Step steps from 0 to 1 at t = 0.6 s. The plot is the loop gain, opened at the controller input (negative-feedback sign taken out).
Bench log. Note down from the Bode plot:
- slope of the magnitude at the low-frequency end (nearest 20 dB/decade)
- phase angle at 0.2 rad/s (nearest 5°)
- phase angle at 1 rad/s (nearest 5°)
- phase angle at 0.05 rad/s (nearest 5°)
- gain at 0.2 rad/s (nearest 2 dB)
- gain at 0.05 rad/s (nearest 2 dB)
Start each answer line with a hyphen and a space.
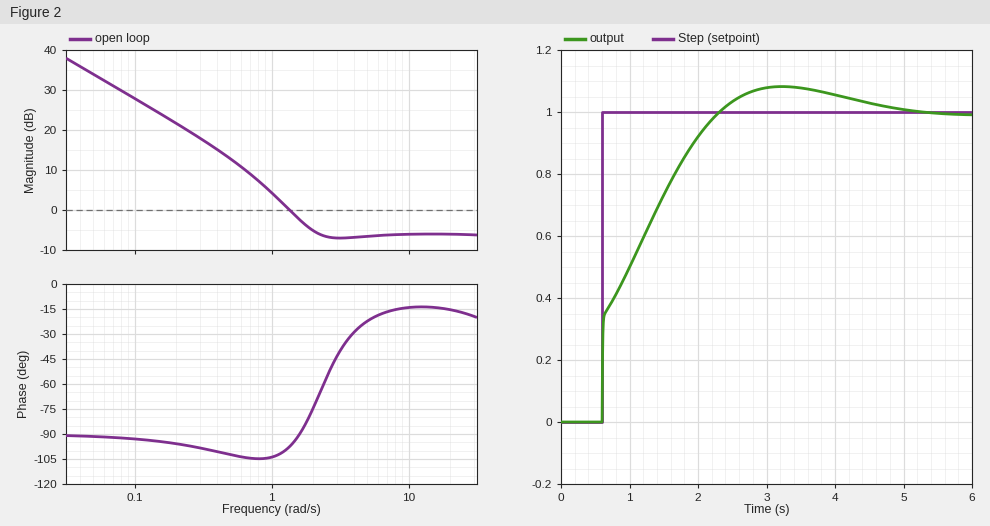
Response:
- -20 dB/decade
- -95°
- -105°
- -90°
- 22 dB
- 34 dB
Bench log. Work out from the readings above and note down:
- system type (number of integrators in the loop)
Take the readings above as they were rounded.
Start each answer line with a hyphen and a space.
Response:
- 1
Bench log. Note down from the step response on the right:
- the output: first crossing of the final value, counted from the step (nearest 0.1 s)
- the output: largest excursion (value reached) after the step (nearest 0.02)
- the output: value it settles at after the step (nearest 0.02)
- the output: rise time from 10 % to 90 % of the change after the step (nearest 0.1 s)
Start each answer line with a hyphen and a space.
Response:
- 1.7 s
- 1.08
- 1.00
- 1.3 s
